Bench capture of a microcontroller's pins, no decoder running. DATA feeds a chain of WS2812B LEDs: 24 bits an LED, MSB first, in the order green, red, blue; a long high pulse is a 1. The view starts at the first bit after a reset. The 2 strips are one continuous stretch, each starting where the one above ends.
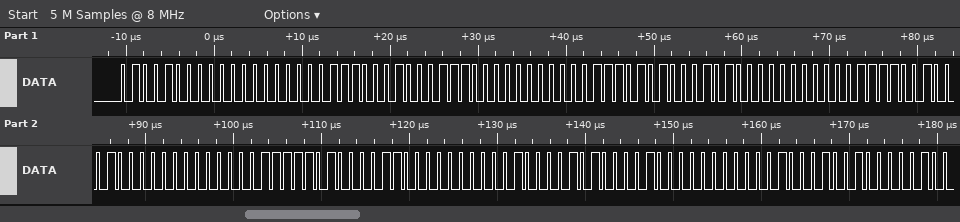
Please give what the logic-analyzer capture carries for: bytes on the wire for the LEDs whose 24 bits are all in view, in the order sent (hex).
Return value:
48 00 1C 47 00 1D 45 00 1E 44 00 1F 43 00 21 42 00 22
